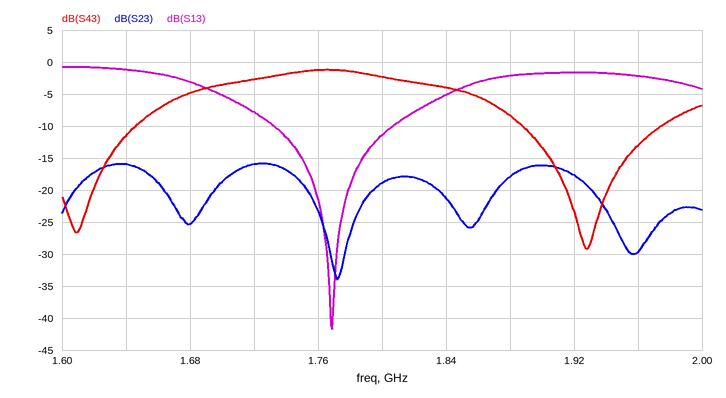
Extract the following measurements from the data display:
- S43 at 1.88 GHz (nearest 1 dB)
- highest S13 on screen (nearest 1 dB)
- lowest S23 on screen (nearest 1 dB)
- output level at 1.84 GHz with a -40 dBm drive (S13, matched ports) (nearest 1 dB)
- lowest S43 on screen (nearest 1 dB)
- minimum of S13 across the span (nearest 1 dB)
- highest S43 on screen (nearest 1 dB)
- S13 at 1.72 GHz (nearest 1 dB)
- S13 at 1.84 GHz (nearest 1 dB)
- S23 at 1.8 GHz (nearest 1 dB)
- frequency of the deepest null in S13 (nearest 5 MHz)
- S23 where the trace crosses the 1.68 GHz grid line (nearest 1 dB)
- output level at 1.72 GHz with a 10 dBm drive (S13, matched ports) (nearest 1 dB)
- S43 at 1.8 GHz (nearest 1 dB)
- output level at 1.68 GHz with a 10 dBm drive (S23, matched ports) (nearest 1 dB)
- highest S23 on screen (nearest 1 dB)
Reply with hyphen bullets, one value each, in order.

- -8 dB
- -1 dB
- -34 dB
- -45 dBm
- -29 dB
- -42 dB
- -1 dB
- -8 dB
- -5 dB
- -19 dB
- 1.770 GHz
- -25 dB
- 2 dBm
- -2 dB
- -15 dBm
- -16 dB
